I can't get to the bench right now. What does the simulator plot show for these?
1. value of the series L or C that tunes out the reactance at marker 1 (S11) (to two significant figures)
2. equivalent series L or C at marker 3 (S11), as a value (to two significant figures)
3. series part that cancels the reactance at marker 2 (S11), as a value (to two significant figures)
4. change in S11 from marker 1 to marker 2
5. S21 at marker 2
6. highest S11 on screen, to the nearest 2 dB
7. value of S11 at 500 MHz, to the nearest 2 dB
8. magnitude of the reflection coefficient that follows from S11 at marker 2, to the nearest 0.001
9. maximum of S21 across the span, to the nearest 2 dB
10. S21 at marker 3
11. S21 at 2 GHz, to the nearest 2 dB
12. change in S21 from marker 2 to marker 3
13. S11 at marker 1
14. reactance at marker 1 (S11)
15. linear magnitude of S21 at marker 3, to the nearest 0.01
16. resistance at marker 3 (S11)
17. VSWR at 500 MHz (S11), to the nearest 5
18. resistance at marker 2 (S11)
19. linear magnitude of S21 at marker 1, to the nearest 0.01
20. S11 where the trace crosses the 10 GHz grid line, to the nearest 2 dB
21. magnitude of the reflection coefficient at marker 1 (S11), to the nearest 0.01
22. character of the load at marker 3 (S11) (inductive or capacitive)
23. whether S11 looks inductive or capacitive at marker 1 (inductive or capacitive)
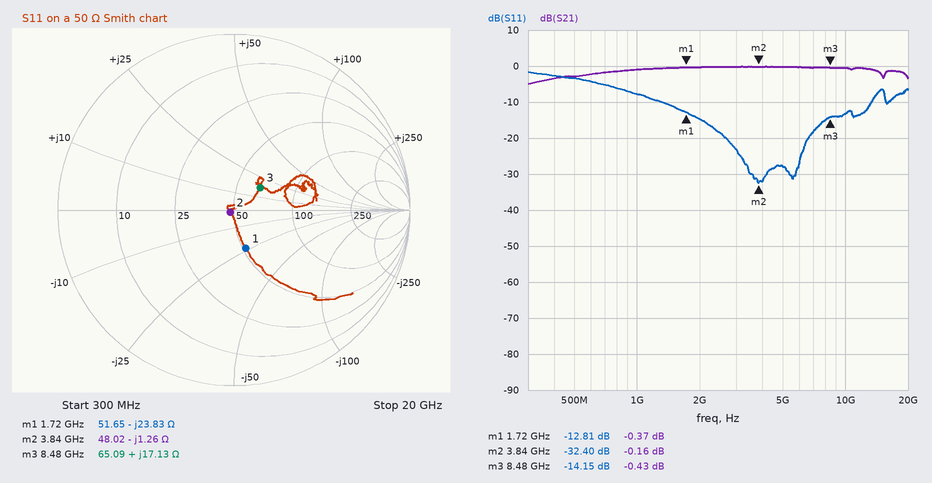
2.2 nH
320 pH
52 pH
-19.59 dB
-0.16 dB
-2 dB
-4 dB
0.024
0 dB
-0.43 dB
0 dB
-0.27 dB
-12.81 dB
-23.83 Ω
0.95
65.09 Ω
5
48.02 Ω
0.96
-14 dB
0.23
inductive
capacitive
